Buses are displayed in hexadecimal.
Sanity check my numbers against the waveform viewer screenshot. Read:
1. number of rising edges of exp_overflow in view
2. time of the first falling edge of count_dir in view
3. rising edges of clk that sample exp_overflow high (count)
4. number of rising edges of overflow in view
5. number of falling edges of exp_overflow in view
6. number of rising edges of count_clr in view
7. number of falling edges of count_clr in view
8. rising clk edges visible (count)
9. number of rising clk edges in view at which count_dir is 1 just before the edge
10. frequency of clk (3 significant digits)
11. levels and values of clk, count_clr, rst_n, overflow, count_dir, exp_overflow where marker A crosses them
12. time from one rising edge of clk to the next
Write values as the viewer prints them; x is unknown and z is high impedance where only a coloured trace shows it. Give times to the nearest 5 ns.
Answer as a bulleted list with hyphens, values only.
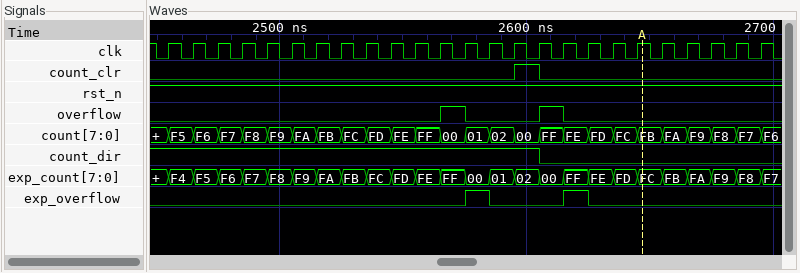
- 2
- 2605 ns
- 2
- 2
- 2
- 1
- 1
- 25
- 16
- 100 MHz
- clk=1, count_clr=0, rst_n=1, overflow=0, count_dir=0, exp_overflow=0
- 10 ns
